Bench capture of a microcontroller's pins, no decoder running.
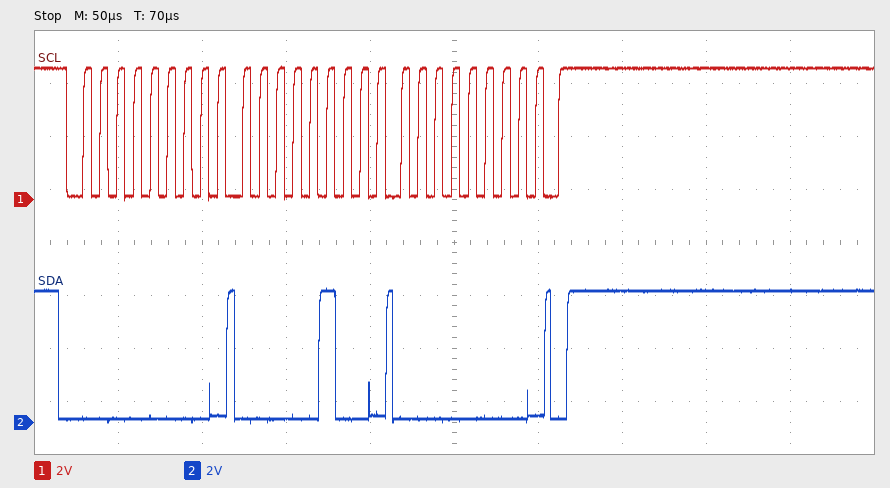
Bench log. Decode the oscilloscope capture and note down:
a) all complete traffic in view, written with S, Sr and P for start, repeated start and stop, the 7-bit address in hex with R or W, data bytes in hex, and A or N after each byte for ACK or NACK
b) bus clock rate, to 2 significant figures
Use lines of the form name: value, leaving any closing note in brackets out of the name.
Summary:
all complete traffic in view, written with S, Sr and P for start, repeated start and stop, the 7-bit address in hex with R or W, data bytes in hex, and A or N after each byte for ACK or NACK: S 00W A 04 A 00 A P
bus clock rate, to 2 significant figures: 100 kHz
